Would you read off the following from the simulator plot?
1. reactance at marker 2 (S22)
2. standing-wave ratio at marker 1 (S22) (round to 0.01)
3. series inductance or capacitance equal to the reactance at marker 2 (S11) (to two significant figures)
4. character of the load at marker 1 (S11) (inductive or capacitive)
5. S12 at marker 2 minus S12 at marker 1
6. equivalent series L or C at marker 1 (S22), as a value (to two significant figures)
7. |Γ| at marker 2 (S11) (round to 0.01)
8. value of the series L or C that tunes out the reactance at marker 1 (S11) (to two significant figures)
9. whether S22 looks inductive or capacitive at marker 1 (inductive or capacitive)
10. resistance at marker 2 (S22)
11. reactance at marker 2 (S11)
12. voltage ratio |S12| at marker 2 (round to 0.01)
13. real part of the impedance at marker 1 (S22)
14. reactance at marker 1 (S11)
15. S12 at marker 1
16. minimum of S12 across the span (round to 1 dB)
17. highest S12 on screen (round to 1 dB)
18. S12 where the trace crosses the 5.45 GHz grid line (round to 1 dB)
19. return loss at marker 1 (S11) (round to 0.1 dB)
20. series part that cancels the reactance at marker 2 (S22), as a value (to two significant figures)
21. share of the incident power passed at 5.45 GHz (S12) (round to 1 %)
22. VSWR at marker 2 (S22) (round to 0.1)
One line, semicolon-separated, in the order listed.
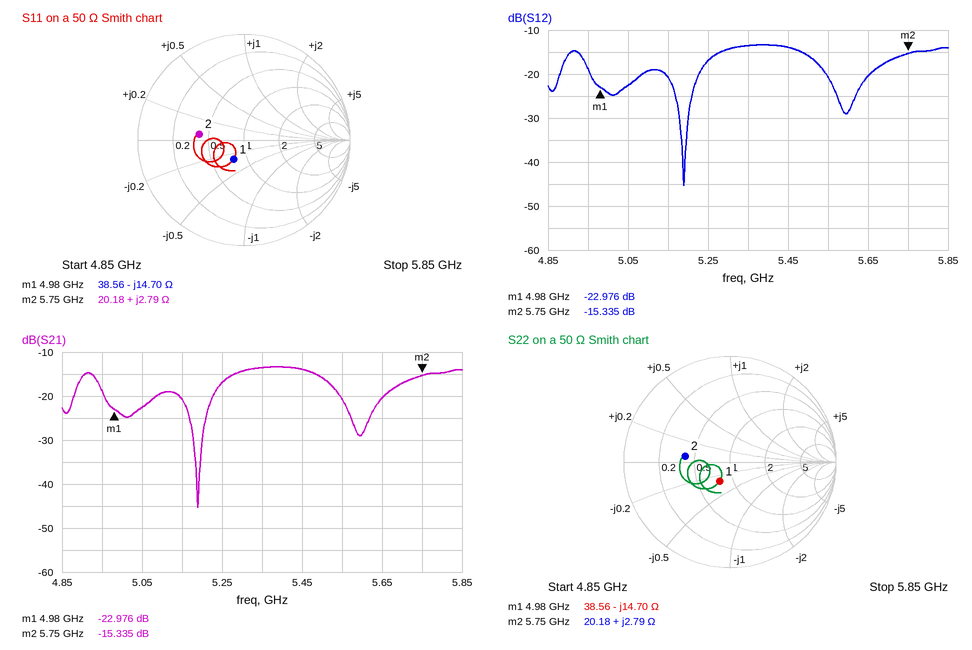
+2.79 Ω; 1.52; 77 pH; capacitive; 7.641 dB; 2.2 pF; 0.43; 470 pH; capacitive; 20.18 Ω; +2.79 Ω; 0.17; 38.56 Ω; -14.70 Ω; -22.976 dB; -45 dB; -13 dB; -14 dB; 13.7 dB; 9.9 pF; 4 %; 2.5
